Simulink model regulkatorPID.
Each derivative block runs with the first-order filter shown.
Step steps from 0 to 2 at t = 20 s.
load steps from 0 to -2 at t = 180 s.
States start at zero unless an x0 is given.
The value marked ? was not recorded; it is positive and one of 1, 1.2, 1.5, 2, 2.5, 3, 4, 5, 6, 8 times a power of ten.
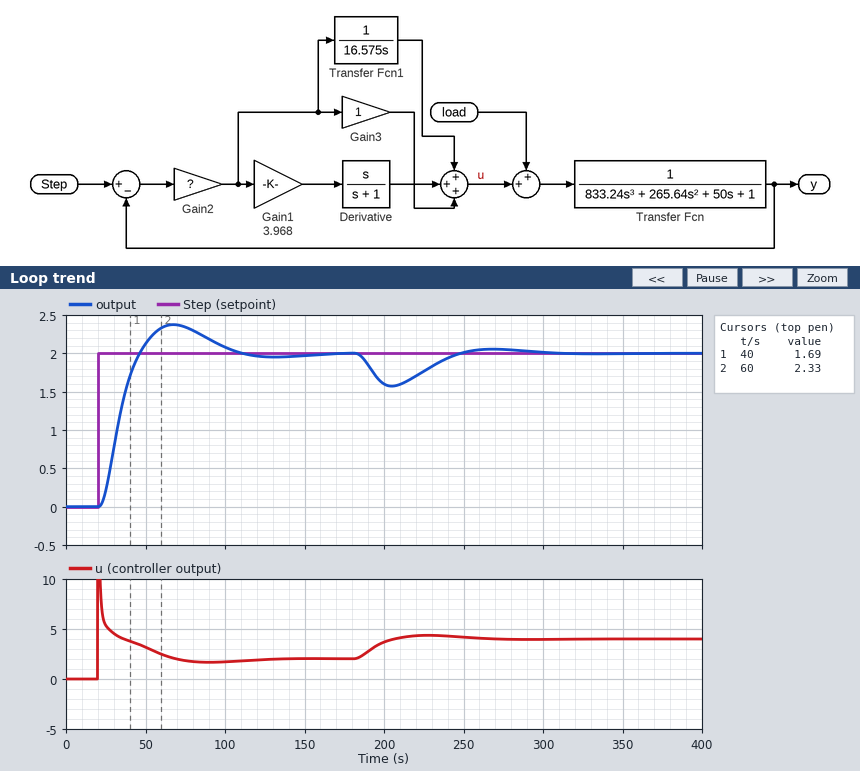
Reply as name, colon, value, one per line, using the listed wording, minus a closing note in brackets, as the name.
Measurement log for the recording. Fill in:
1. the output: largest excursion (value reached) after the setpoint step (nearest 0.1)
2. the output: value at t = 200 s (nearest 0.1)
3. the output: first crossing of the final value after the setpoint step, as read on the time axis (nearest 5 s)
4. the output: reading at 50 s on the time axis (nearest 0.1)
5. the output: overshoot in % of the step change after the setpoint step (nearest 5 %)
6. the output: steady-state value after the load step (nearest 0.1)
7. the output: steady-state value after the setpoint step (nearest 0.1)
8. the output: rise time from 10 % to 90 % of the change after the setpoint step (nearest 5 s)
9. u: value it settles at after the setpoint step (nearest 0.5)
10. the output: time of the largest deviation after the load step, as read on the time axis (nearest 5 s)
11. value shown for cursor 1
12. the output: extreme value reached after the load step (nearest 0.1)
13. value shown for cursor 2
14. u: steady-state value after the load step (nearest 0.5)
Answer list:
the output: largest excursion (value reached) after the setpoint step: 2.4
the output: value at t = 200 s: 1.6
the output: first crossing of the final value after the setpoint step, as read on the time axis: 45 s
the output: reading at 50 s on the time axis: 2.1
the output: overshoot in % of the step change after the setpoint step: 20 %
the output: steady-state value after the load step: 2.0
the output: steady-state value after the setpoint step: 2.0
the output: rise time from 10 % to 90 % of the change after the setpoint step: 15 s
u: value it settles at after the setpoint step: 2.0
the output: time of the largest deviation after the load step, as read on the time axis: 205 s
value shown for cursor 1: 1.69
the output: extreme value reached after the load step: 1.6
value shown for cursor 2: 2.33
u: steady-state value after the load step: 4.0
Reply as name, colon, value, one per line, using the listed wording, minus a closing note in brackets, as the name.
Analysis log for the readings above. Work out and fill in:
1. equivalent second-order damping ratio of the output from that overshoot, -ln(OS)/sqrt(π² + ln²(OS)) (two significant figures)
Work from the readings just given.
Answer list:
equivalent second-order damping ratio of the output from that overshoot, -ln(OS)/sqrt(π² + ln²(OS)): 0.46
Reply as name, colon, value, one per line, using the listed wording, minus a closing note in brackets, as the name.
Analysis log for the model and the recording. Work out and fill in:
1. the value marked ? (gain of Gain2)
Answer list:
the value marked ?: 2.5
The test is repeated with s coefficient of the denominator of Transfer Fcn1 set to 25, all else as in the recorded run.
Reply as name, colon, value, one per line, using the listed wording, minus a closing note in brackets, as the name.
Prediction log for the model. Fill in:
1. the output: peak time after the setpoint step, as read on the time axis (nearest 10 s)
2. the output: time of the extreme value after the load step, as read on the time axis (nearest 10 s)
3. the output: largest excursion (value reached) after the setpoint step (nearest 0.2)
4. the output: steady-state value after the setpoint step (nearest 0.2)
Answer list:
the output: peak time after the setpoint step, as read on the time axis: 80 s
the output: time of the extreme value after the load step, as read on the time axis: 210 s
the output: largest excursion (value reached) after the setpoint step: 2.2
the output: steady-state value after the setpoint step: 2.0
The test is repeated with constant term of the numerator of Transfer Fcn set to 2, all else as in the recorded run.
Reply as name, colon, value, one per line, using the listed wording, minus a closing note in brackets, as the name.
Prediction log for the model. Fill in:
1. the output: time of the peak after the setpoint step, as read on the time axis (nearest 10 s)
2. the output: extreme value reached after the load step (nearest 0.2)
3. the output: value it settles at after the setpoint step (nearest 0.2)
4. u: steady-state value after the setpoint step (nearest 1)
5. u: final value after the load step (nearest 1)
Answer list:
the output: time of the peak after the setpoint step, as read on the time axis: 40 s
the output: extreme value reached after the load step: 1.4
the output: value it settles at after the setpoint step: 2.0
u: steady-state value after the setpoint step: 1
u: final value after the load step: 3
